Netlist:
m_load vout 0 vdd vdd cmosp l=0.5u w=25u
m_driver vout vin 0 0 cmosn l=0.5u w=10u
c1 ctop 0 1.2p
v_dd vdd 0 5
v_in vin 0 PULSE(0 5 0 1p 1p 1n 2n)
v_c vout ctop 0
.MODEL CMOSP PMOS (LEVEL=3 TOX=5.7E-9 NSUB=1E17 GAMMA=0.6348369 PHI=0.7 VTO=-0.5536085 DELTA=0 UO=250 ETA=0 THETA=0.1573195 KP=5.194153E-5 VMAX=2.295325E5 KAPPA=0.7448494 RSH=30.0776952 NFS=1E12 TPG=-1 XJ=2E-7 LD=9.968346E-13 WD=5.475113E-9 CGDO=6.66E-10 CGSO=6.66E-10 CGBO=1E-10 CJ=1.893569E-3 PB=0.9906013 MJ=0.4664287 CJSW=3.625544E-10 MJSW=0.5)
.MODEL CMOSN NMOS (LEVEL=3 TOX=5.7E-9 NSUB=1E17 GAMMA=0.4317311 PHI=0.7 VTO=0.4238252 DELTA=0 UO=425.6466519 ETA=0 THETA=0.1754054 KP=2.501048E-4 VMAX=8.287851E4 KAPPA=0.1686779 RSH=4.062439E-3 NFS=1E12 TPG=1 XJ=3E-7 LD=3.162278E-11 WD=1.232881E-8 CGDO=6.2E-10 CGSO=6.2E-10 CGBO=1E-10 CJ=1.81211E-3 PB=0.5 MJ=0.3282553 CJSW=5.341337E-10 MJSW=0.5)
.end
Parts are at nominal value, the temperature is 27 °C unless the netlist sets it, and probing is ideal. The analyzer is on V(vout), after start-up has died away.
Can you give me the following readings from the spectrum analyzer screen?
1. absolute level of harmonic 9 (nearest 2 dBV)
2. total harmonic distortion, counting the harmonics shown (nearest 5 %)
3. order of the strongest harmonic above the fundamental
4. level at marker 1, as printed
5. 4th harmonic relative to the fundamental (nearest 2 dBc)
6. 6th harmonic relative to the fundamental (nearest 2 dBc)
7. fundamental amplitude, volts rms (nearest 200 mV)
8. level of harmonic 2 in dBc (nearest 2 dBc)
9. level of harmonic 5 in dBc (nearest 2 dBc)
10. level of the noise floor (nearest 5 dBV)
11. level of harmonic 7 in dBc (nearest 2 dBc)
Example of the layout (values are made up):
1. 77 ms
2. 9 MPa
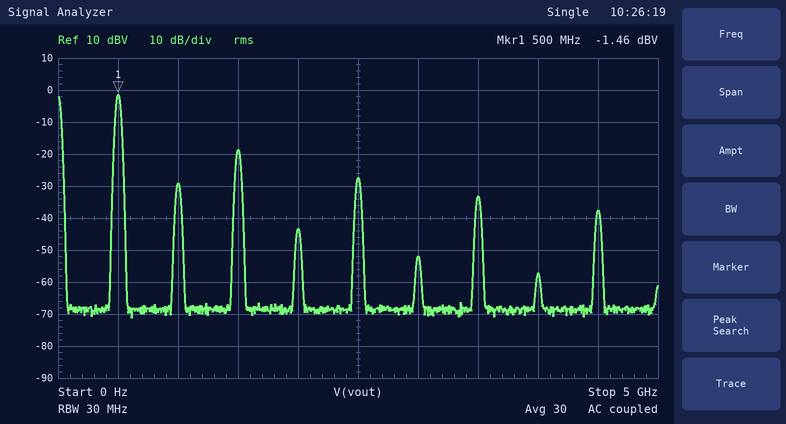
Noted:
1. -38 dBV
2. 15 %
3. 3
4. -1.46 dBV
5. -42 dBc
6. -50 dBc
7. 800 mV
8. -28 dBc
9. -26 dBc
10. -70 dBV
11. -32 dBc
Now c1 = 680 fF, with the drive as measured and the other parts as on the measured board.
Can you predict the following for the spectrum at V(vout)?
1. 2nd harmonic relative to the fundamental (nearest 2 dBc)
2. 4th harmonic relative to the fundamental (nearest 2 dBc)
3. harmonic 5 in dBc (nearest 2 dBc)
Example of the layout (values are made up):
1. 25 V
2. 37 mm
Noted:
1. -24 dBc
2. -36 dBc
3. -24 dBc
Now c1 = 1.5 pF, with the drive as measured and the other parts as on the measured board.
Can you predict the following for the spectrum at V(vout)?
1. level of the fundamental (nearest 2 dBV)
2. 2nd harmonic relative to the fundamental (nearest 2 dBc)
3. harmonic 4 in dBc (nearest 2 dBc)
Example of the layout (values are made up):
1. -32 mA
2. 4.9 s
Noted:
1. -2 dBV
2. -30 dBc
3. -44 dBc
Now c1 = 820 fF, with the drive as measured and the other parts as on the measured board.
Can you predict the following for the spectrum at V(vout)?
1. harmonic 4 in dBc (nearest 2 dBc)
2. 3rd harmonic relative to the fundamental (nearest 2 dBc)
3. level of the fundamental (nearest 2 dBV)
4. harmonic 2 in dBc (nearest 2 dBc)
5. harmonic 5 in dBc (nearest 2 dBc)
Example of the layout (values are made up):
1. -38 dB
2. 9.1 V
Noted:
1. -38 dBc
2. -16 dBc
3. 0 dBV
4. -24 dBc
5. -24 dBc
